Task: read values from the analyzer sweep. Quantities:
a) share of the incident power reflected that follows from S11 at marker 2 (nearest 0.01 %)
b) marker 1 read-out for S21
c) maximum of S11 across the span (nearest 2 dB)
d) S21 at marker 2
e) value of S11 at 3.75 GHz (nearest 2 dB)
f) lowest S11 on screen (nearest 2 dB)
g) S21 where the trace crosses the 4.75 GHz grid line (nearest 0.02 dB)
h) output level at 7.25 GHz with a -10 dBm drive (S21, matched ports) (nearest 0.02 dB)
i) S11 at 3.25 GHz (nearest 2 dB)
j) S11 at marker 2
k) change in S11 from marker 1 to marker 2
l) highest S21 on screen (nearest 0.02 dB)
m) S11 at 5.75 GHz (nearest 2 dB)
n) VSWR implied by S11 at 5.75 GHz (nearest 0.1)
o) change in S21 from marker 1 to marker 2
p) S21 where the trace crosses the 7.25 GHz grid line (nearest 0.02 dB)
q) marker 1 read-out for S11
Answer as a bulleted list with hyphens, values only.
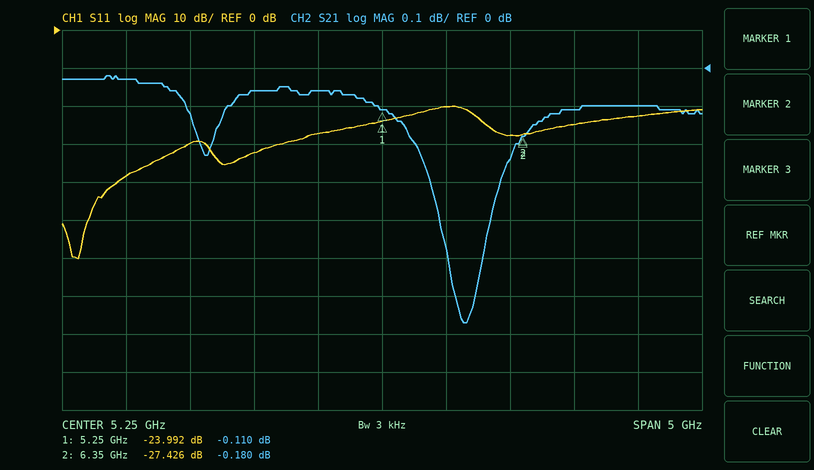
- 0.18 %
- -0.110 dB
- -20 dB
- -0.180 dB
- -30 dB
- -60 dB
- -0.06 dB
- -10.10 dBm
- -38 dB
- -27.426 dB
- -3.434 dB
- -0.02 dB
- -20 dB
- 1.2
- -0.070 dB
- -0.10 dB
- -23.992 dB
